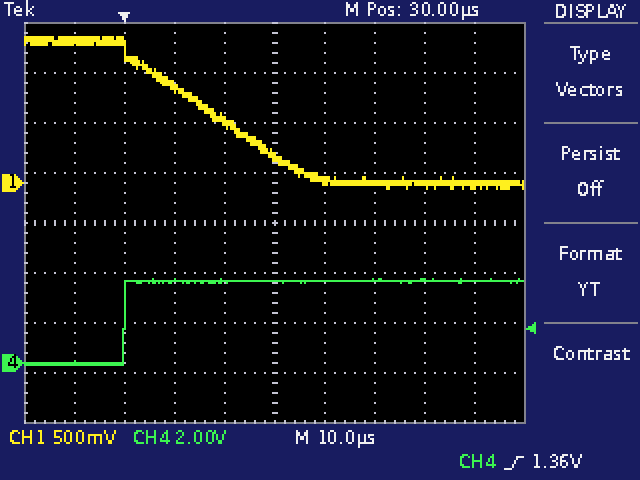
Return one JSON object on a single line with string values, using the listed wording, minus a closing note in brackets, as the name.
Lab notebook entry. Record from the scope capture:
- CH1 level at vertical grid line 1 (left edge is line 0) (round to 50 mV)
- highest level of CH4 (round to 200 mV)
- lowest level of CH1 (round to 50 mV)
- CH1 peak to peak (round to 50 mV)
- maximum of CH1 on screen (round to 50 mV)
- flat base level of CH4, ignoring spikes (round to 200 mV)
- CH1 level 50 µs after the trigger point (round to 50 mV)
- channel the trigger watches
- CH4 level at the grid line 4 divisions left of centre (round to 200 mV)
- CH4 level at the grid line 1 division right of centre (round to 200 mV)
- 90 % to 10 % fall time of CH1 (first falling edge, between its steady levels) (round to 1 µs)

{"CH1 level at vertical grid line 1 (left edge is line 0)": "1.40 V", "highest level of CH4": "3.4 V", "lowest level of CH1": "-50 mV", "CH1 peak to peak": "1.50 V", "maximum of CH1 on screen": "1.45 V", "flat base level of CH4, ignoring spikes": "0.0 V", "CH1 level 50 µs after the trigger point": "0 mV", "channel the trigger watches": "CH4", "CH4 level at the grid line 4 divisions left of centre": "0.0 V", "CH4 level at the grid line 1 division right of centre": "3.2 V", "90 % to 10 % fall time of CH1 (first falling edge, between its steady levels)": "34 µs"}
